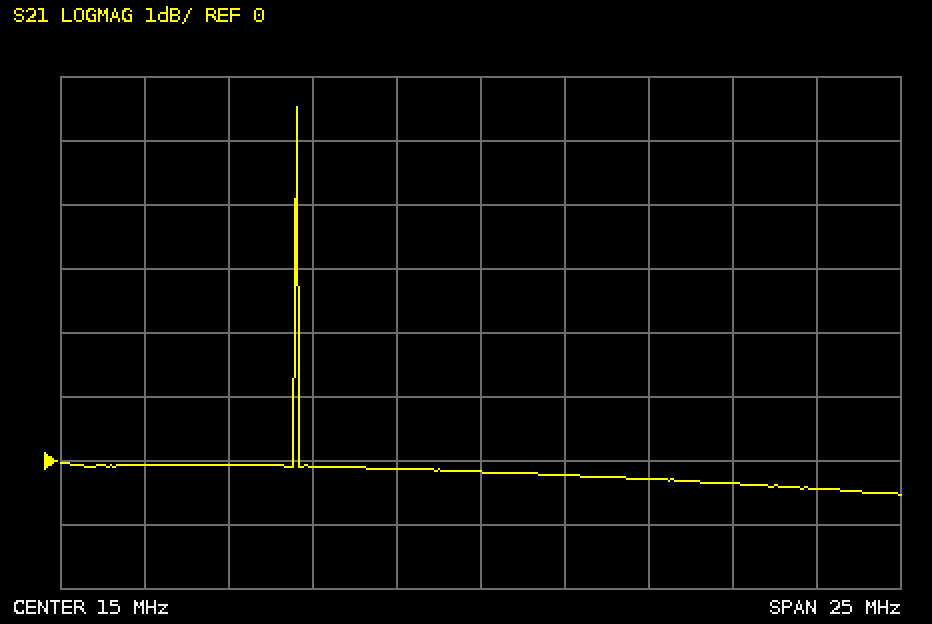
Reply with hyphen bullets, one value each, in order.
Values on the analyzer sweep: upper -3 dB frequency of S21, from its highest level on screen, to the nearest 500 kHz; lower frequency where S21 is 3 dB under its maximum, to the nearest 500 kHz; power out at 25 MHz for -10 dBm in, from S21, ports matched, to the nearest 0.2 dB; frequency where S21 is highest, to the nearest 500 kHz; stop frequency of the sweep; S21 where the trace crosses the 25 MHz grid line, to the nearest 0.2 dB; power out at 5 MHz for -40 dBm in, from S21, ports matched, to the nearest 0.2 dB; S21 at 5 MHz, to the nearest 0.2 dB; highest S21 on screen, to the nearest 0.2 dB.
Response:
- 9.5 MHz
- 9.5 MHz
- -10.4 dBm
- 9.5 MHz
- 27.5 MHz
- -0.4 dB
- -40.0 dBm
- 0.0 dB
- 5.6 dB
